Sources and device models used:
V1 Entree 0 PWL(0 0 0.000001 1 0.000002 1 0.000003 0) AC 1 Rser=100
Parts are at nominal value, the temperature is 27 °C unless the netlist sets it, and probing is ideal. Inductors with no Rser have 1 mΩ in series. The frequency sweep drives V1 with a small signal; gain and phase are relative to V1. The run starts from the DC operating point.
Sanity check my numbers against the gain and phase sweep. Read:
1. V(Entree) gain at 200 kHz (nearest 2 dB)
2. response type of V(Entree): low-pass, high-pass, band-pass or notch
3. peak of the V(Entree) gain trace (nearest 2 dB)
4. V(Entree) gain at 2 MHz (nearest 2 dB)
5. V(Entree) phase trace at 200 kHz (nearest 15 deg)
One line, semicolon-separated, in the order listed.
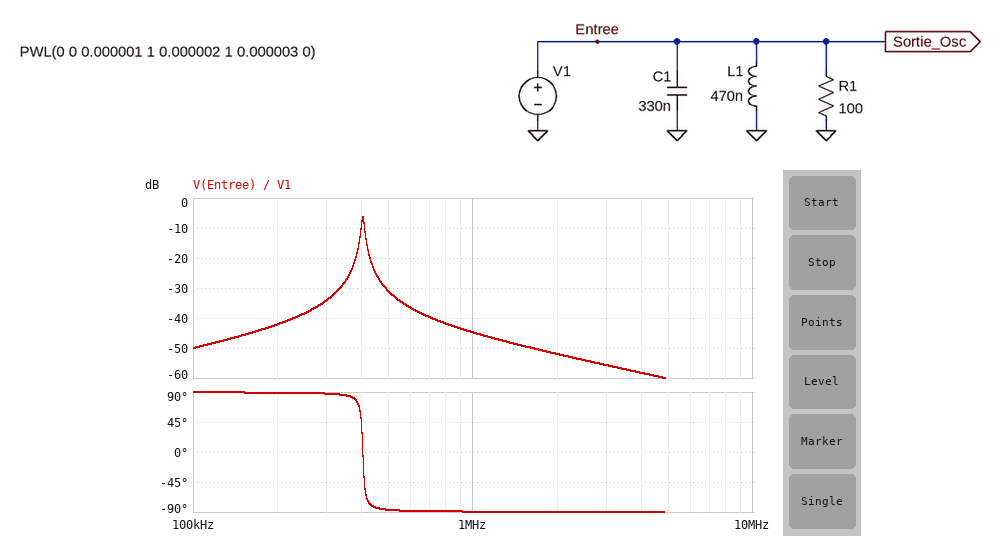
-42 dB; band-pass; -6 dB; -52 dB; 90 deg
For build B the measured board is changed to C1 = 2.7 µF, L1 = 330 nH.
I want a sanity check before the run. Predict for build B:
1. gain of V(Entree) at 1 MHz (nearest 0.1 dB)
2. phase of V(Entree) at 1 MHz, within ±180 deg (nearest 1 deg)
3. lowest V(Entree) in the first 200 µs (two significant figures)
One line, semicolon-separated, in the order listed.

-64.3 dB; -90 deg; -5.7 mV
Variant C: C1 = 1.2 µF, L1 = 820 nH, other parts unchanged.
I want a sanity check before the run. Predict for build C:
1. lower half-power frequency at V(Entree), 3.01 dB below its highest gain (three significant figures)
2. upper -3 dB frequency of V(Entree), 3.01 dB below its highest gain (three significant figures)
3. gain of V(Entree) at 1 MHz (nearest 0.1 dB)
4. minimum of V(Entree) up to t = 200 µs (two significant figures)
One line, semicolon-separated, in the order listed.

159 kHz; 162 kHz; -57.3 dB; -13 mV
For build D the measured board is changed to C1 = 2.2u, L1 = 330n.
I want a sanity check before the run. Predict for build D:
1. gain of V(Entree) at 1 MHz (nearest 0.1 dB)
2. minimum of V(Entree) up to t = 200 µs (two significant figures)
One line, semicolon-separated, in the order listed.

-62.5 dB; -6.6 mV
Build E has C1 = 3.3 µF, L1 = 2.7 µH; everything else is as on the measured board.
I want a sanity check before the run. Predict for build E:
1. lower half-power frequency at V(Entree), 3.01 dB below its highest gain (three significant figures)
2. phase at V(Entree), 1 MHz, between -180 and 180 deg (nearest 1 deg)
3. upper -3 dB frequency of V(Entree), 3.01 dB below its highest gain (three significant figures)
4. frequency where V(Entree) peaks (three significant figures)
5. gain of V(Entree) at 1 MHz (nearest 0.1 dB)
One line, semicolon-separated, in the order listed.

52.8 kHz; -90 deg; 53.8 kHz; 53.3 kHz; -66.3 dB
